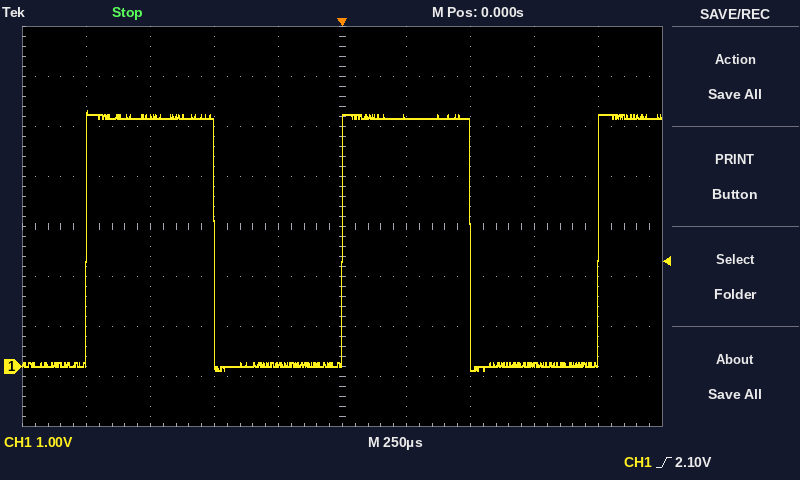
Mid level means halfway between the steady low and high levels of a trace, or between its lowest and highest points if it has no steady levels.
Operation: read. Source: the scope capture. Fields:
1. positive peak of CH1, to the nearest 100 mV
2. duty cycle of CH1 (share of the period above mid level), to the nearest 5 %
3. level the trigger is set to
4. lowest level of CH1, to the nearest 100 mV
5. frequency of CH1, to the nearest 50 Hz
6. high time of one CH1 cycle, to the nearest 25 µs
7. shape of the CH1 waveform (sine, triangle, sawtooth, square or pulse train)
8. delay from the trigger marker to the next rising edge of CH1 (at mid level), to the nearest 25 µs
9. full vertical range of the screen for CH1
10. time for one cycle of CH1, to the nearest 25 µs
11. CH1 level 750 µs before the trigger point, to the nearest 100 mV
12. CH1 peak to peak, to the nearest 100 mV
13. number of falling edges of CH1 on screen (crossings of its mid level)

5.1 V
50 %
2.10 V
-100 mV
1.00 kHz
500 µs
square
1.000 ms
8 V
1.000 ms
5.0 V
5.2 V
2
